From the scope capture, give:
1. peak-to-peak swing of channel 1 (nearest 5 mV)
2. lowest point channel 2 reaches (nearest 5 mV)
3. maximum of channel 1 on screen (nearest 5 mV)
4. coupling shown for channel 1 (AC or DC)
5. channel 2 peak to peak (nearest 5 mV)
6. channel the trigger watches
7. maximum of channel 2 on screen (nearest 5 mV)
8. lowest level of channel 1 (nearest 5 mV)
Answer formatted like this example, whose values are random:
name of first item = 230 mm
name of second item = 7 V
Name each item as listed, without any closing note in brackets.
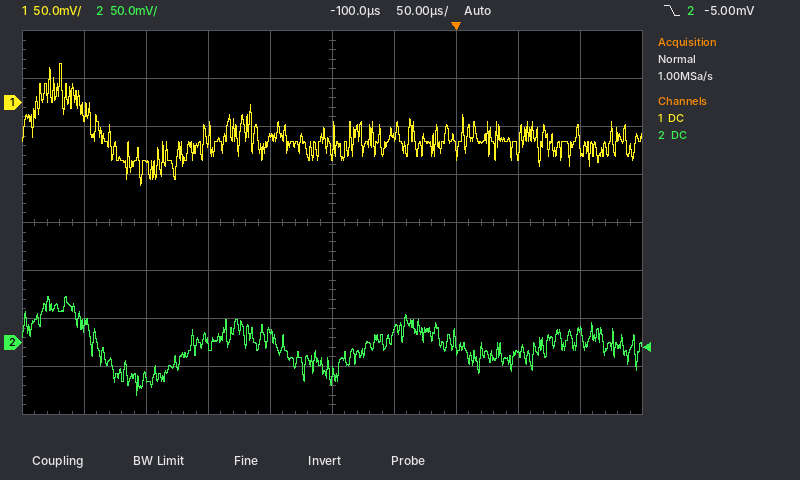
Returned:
peak-to-peak swing of channel 1 = 125 mV
lowest point channel 2 reaches = -55 mV
maximum of channel 1 on screen = 40 mV
coupling shown for channel 1 = DC
channel 2 peak to peak = 105 mV
channel the trigger watches = channel 2
maximum of channel 2 on screen = 50 mV
lowest level of channel 1 = -85 mV
